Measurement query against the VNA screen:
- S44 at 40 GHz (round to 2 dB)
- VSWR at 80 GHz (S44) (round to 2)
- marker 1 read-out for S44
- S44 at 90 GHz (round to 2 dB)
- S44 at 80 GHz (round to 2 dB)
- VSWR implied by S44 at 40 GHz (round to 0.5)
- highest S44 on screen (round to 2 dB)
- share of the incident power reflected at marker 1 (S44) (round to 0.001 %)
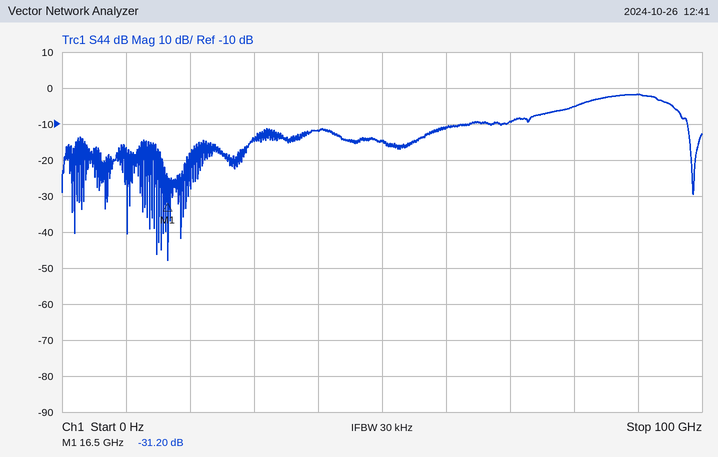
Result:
-12 dB
4
-31.20 dB
-2 dB
-6 dB
1.5
-2 dB
0.076 %
